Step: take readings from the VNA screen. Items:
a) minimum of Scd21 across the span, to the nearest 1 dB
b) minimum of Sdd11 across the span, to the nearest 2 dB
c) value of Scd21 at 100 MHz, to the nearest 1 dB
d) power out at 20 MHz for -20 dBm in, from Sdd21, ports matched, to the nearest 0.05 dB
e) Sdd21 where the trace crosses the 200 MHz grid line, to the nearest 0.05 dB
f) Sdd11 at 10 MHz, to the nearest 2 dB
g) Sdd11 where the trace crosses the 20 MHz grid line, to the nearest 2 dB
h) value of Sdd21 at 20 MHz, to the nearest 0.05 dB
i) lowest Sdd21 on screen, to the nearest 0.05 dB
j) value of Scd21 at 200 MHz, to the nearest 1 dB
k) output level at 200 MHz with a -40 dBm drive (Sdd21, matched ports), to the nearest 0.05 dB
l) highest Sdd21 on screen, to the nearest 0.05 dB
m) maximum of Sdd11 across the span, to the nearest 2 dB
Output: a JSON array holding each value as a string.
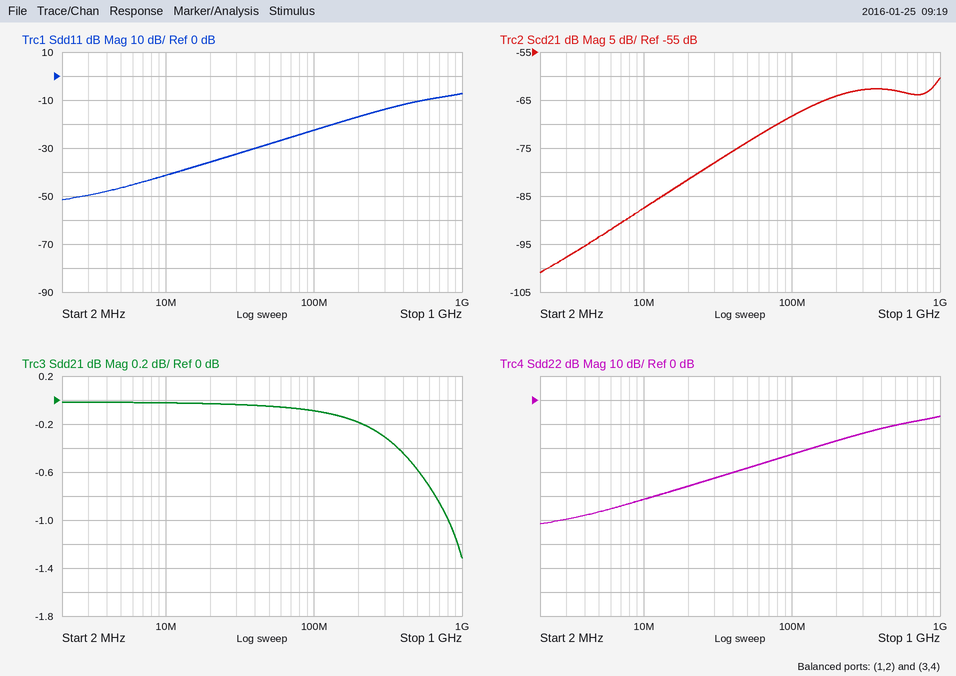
["-101 dB", "-52 dB", "-68 dB", "-20.05 dBm", "-0.20 dB", "-42 dB", "-36 dB", "-0.05 dB", "-1.30 dB", "-64 dB", "-40.20 dBm", "0.00 dB", "-8 dB"]
